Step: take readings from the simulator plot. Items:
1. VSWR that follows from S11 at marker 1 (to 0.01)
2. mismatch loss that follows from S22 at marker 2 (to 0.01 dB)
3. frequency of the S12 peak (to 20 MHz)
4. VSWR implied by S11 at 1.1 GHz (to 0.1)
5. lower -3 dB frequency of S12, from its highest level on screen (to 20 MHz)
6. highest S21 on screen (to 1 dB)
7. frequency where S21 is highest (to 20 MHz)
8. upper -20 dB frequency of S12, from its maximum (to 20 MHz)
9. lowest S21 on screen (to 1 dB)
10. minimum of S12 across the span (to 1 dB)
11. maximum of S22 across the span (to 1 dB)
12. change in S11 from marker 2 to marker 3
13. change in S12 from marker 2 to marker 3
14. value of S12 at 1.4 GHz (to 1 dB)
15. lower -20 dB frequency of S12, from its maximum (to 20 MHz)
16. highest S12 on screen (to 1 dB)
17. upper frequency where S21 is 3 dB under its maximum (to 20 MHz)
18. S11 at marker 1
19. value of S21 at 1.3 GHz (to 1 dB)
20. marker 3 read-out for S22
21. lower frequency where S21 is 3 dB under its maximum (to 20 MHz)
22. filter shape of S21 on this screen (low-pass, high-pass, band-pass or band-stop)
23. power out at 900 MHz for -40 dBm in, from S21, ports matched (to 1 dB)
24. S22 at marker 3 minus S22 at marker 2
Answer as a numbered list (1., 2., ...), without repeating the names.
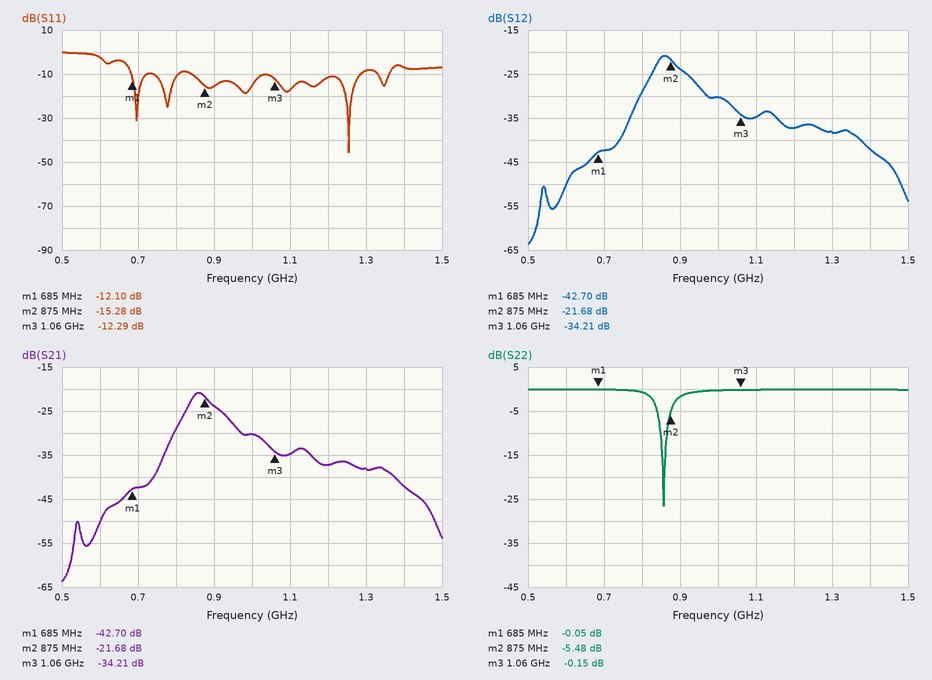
1. 1.66
2. 1.45 dB
3. 860 MHz
4. 1.3
5. 840 MHz
6. -21 dB
7. 860 MHz
8. 1.38 GHz
9. -64 dB
10. -64 dB
11. 0 dB
12. 2.99 dB
13. -12.53 dB
14. -42 dB
15. 740 MHz
16. -21 dB
17. 900 MHz
18. -12.10 dB
19. -38 dB
20. -0.15 dB
21. 840 MHz
22. band-pass
23. -64 dBm
24. 5.33 dB
